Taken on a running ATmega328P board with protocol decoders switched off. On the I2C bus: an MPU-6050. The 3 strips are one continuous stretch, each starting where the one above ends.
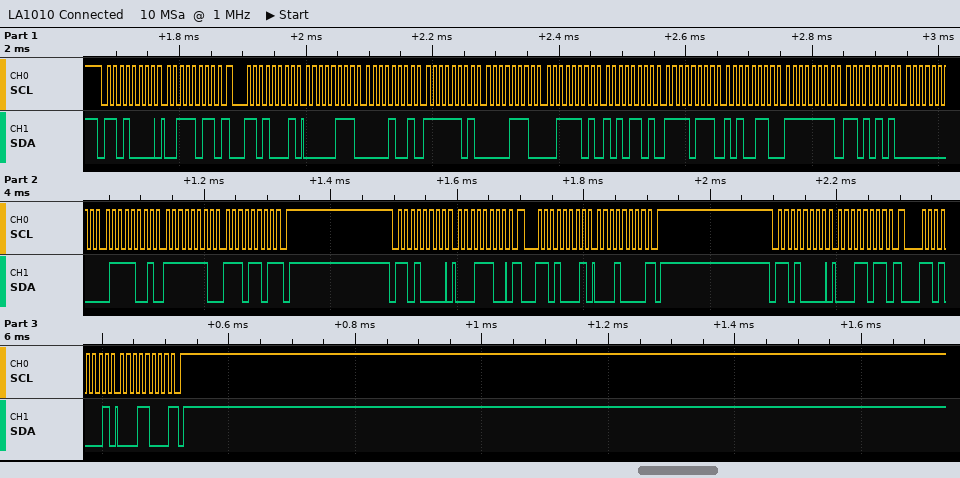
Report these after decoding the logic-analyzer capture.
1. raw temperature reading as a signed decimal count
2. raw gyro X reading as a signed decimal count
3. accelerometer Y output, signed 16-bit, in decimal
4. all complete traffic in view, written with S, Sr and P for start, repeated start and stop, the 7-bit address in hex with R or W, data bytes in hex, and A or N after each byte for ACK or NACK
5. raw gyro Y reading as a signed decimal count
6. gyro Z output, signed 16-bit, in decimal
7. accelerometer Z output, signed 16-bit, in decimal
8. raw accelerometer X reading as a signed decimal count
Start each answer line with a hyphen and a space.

- -2138
- -43
- -754
- S 68W A 3B A Sr 68R A 07 A 09 A FD A 0E A 3D A AD A F7 A A6 A FF A D5 A 00 A 79 A FE A ED N P S 68W A 1C A Sr 68R A 10 N P S 68W A 1B A Sr 68R A 18 N P
- 121
- -275
- 15789
- 1801
